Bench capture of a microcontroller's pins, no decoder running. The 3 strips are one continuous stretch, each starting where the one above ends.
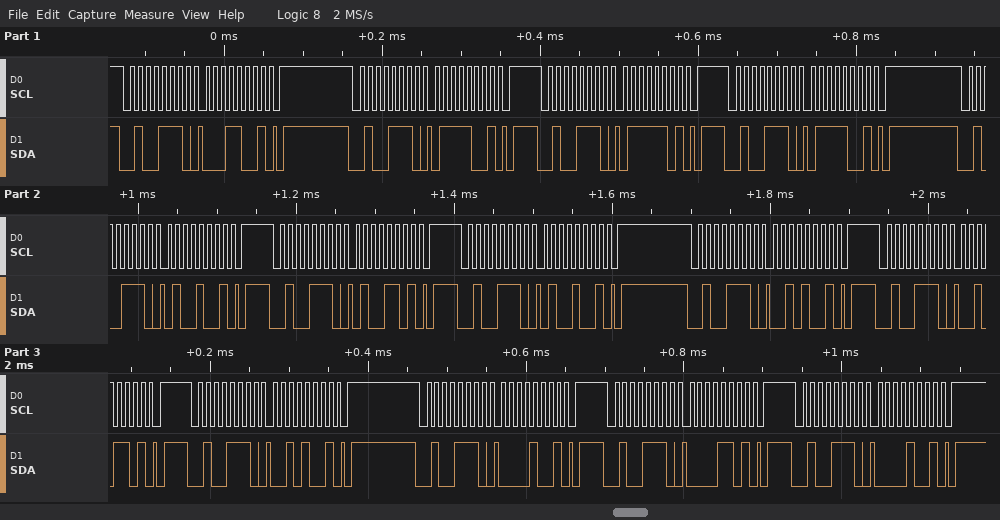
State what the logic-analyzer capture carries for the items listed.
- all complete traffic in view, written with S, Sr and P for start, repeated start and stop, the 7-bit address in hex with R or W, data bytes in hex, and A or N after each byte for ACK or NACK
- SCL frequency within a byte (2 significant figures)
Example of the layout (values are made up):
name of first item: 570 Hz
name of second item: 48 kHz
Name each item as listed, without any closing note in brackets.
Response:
all complete traffic in view, written with S, Sr and P for start, repeated start and stop, the 7-bit address in hex with R or W, data bytes in hex, and A or N after each byte for ACK or NACK: S 27W A 19 A P S 27W A 79 A P S 27W A 7D A P S 27W A 79 A P S 27W A 49 A P S 27W A 4D A P S 27W A 49 A P S 27W A 29 A P S 27W A 2D A P S 27W A 29 A P S 27W A 09 A P S 27W A 0D A P S 27W A 09 A P
SCL frequency within a byte: 100 kHz
